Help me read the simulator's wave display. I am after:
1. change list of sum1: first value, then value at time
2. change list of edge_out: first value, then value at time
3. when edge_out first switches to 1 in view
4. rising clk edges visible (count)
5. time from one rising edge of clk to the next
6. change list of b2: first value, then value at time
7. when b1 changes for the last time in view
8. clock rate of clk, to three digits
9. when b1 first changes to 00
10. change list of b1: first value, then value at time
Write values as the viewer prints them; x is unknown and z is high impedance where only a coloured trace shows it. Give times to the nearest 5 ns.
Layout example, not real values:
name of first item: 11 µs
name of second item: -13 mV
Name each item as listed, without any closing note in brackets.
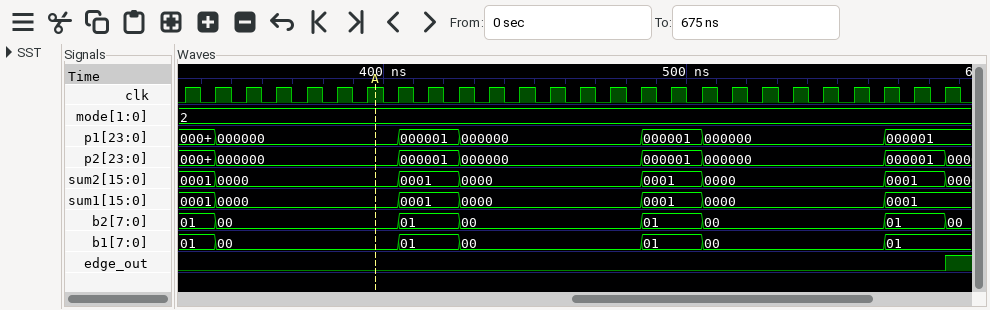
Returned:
change list of sum1: first value, then value at time: 0001, 0000 at 345 ns, 0001 at 405 ns, 0000 at 425 ns, 0001 at 485 ns, 0000 at 505 ns, 0001 at 565 ns
change list of edge_out: first value, then value at time: 0, 1 at 585 ns
when edge_out first switches to 1 in view: 585 ns
rising clk edges visible: 26
time from one rising edge of clk to the next: 10 ns
change list of b2: first value, then value at time: 01, 00 at 345 ns, 01 at 405 ns, 00 at 425 ns, 01 at 485 ns, 00 at 505 ns, 01 at 565 ns, 00 at 585 ns
when b1 changes for the last time in view: 565 ns
clock rate of clk, to three digits: 100 MHz
when b1 first changes to 00: 345 ns
change list of b1: first value, then value at time: 01, 00 at 345 ns, 01 at 405 ns, 00 at 425 ns, 01 at 485 ns, 00 at 505 ns, 01 at 565 ns
